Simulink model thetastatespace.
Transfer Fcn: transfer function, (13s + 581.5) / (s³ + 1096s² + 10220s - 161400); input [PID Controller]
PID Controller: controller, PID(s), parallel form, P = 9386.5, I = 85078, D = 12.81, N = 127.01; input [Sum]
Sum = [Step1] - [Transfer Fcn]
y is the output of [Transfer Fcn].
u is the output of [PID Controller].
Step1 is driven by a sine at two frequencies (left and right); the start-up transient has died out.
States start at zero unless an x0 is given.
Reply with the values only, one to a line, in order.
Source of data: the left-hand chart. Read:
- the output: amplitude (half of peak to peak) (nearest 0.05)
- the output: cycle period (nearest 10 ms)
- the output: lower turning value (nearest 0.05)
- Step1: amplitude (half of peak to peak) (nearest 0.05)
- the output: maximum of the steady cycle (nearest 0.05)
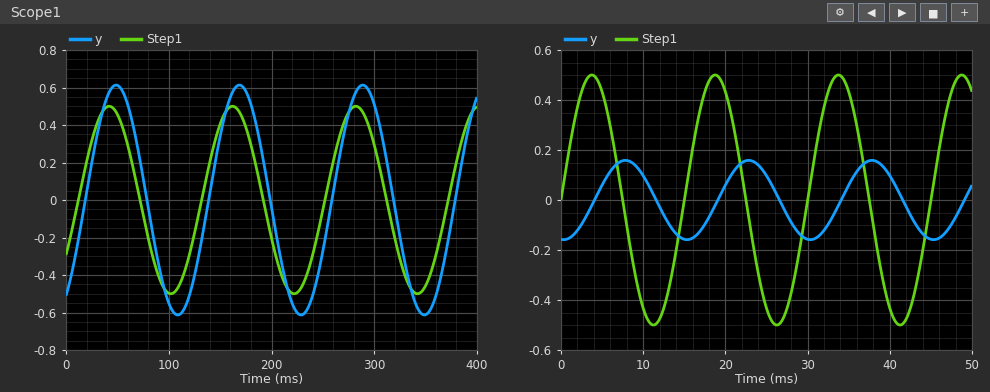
0.60
120 ms
-0.60
0.50
0.60
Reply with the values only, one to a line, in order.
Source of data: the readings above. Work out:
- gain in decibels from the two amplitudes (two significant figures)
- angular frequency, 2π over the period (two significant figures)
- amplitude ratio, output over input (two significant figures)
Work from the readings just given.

1.6 dB
0.052 rad/ms
1.2
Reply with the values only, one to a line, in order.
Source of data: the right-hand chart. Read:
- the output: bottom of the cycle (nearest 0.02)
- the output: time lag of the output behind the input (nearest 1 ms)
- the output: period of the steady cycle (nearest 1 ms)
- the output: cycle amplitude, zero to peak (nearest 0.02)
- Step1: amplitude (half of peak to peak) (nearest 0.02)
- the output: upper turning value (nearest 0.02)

-0.16
4 ms
15 ms
0.16
0.50
0.16
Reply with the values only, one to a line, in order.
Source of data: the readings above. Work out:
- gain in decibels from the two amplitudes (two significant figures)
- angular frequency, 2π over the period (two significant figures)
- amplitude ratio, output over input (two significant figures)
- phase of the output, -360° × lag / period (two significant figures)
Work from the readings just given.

-9.9 dB
0.42 rad/ms
0.32
-96°
